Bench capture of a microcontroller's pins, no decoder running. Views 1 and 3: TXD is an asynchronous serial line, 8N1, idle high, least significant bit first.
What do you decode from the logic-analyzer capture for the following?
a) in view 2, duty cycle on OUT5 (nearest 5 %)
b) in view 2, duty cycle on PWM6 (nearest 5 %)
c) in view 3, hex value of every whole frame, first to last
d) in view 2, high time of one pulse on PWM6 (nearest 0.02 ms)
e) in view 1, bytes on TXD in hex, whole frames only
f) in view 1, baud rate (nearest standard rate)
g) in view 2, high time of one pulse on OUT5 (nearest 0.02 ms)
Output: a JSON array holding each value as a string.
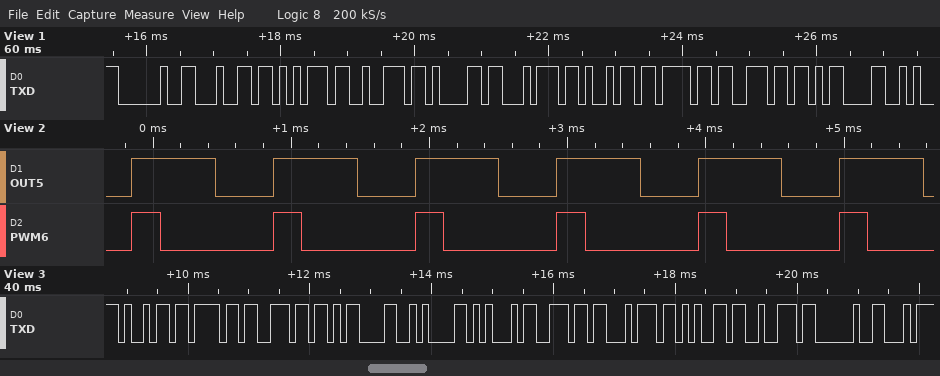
["60 %", "20 %", "69 6F 6E 0D 0A 45 6E 74 65 72 20", "0.20 ms", "20 64 75 72 61 74 69 6F 6E 0D", "9600 baud", "0.60 ms"]
